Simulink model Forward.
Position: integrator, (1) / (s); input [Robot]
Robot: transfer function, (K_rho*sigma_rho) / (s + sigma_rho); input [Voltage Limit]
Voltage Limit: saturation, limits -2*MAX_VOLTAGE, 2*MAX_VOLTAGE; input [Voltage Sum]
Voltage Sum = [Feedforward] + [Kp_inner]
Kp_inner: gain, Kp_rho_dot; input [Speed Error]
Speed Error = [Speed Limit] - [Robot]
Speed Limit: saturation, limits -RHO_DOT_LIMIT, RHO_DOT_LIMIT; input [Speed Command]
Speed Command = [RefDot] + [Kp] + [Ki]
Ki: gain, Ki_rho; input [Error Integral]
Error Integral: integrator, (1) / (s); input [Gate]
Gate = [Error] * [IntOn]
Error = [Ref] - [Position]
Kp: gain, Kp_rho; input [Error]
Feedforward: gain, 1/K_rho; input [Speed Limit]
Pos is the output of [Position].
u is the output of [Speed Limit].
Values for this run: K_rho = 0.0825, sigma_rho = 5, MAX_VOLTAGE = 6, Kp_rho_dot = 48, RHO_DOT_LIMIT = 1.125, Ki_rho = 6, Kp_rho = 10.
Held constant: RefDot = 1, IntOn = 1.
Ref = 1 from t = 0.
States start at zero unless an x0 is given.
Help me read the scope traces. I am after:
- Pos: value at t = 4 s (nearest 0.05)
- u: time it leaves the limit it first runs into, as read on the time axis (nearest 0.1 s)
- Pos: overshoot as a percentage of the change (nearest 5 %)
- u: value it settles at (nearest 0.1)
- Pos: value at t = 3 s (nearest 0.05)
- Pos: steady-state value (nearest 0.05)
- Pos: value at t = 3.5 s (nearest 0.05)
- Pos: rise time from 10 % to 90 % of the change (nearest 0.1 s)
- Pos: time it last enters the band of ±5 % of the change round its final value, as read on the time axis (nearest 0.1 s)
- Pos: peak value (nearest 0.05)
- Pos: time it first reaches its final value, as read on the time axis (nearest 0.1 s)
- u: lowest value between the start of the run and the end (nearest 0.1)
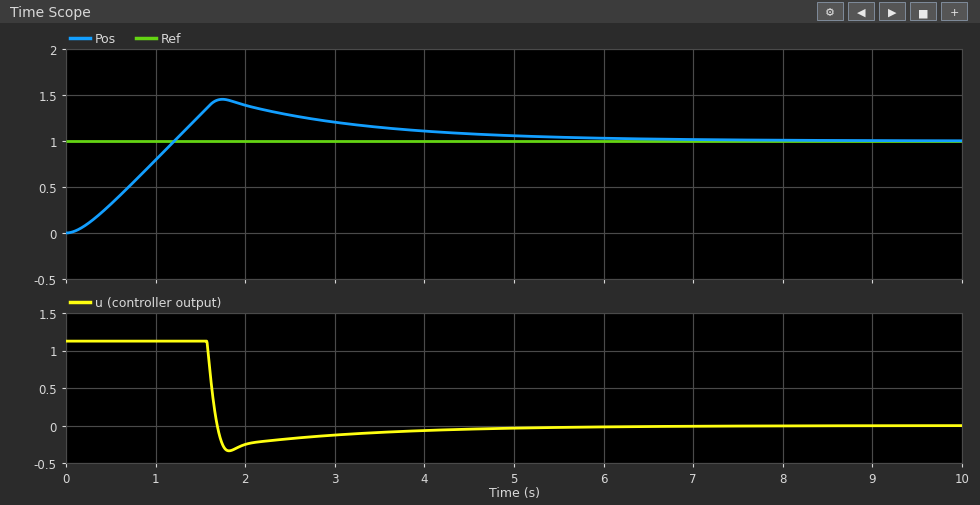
1.10
1.6 s
45 %
0.0
1.20
1.00
1.15
0.9 s
5.2 s
1.45
1.2 s
-0.3
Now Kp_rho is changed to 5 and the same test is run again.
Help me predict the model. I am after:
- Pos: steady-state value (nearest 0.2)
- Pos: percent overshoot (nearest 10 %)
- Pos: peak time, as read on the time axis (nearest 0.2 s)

1.0
70 %
2.0 s
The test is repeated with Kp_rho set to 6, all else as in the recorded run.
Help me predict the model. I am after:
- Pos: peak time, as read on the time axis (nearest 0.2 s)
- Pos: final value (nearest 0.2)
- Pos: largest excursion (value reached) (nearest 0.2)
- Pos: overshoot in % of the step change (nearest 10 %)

2.0 s
1.0
1.6
60 %
